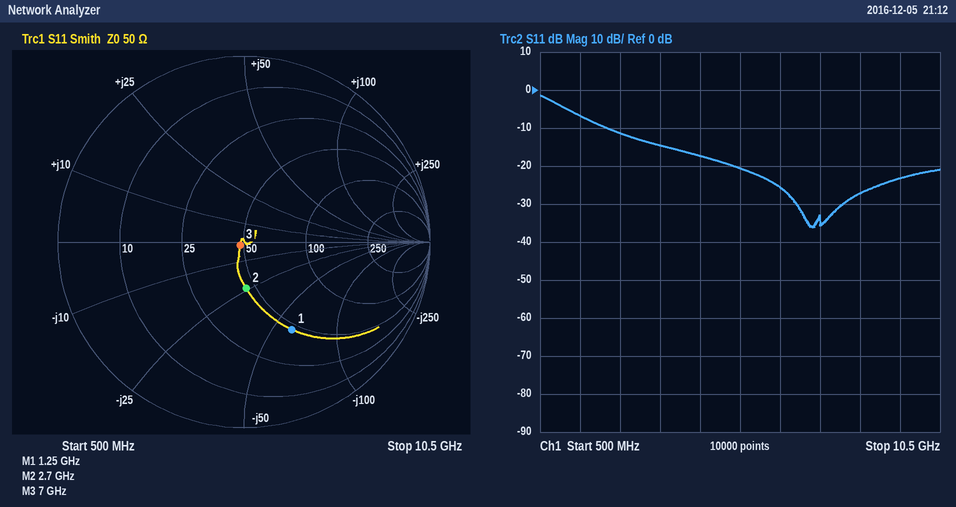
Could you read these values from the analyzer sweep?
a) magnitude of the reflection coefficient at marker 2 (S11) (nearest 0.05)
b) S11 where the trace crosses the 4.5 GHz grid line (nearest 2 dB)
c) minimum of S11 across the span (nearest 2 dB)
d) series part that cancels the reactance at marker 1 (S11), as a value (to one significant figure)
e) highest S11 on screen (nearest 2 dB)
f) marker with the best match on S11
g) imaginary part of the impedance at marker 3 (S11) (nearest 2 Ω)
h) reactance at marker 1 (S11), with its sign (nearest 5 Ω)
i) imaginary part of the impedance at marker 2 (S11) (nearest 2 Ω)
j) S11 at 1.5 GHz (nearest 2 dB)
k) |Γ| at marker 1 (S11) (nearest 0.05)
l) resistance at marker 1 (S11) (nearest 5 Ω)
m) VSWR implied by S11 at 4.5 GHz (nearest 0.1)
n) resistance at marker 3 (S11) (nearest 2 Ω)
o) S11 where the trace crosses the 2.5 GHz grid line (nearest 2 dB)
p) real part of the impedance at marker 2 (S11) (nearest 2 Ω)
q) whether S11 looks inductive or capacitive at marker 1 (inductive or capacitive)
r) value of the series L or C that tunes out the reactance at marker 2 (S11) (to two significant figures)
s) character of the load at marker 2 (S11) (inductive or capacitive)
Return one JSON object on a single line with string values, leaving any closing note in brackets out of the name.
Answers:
{"magnitude of the reflection coefficient at marker 2 (S11)": "0.25", "S11 where the trace crosses the 4.5 GHz grid line": "-18 dB", "minimum of S11 across the span": "-36 dB", "series part that cancels the reactance at marker 1 (S11), as a value": "8 nH", "highest S11 on screen": "-2 dB", "marker with the best match on S11": "marker 3", "imaginary part of the impedance at marker 3 (S11)": "-2 Ω", "reactance at marker 1 (S11), with its sign": "-60 Ω", "imaginary part of the impedance at marker 2 (S11)": "-24 Ω", "S11 at 1.5 GHz": "-6 dB", "|Γ| at marker 1 (S11)": "0.55", "resistance at marker 1 (S11)": "45 Ω", "VSWR implied by S11 at 4.5 GHz": "1.3", "resistance at marker 3 (S11)": "48 Ω", "S11 where the trace crosses the 2.5 GHz grid line": "-12 dB", "real part of the impedance at marker 2 (S11)": "46 Ω", "whether S11 looks inductive or capacitive at marker 1": "capacitive", "value of the series L or C that tunes out the reactance at marker 2 (S11)": "1.4 nH", "character of the load at marker 2 (S11)": "capacitive"}
